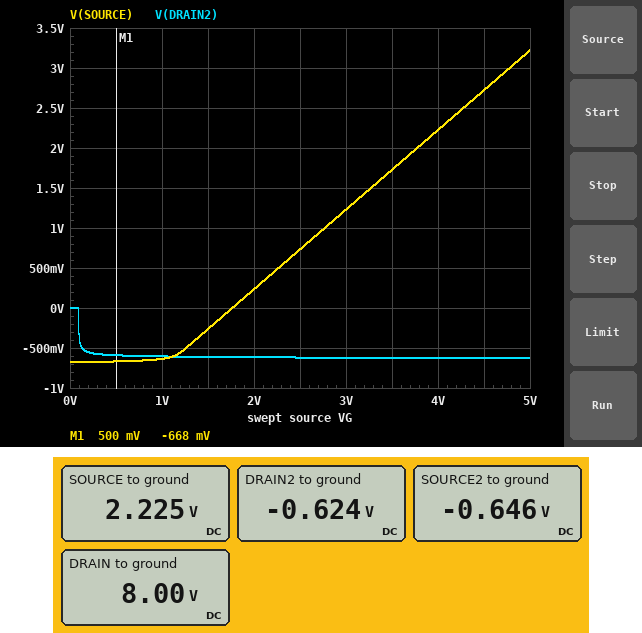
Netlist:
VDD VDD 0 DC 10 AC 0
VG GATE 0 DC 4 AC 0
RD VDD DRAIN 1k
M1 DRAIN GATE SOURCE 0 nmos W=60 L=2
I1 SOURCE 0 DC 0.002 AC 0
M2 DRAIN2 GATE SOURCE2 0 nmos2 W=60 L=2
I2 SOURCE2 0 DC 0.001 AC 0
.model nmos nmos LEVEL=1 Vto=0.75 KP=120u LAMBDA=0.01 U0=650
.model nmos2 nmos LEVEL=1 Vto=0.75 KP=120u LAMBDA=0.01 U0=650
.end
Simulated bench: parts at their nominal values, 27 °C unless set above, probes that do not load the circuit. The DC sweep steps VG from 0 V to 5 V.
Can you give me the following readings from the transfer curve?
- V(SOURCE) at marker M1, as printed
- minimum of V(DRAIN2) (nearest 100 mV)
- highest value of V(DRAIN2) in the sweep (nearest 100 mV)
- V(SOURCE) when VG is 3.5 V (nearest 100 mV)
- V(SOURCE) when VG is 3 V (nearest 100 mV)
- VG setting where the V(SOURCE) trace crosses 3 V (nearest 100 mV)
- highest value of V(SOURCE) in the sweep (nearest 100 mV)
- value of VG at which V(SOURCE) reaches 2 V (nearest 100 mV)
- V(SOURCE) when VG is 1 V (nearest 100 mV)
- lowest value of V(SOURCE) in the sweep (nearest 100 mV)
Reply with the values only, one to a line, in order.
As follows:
-668 mV
-600 mV
0 V
1.7 V
1.2 V
4.8 V
3.2 V
3.8 V
-600 mV
-700 mV
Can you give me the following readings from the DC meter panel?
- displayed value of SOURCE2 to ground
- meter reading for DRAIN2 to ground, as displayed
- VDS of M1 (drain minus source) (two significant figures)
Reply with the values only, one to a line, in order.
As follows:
-0.646 V
-0.624 V
5.8 V
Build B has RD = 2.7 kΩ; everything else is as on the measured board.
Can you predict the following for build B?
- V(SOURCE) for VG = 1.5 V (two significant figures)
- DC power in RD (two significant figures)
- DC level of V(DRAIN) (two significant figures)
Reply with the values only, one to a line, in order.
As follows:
-280 mV
11 mW
4.6 V
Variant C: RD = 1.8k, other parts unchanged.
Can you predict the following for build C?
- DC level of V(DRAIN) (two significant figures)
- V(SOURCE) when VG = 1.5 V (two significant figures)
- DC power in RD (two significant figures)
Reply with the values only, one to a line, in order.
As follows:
6.4 V
-270 mV
7.2 mW
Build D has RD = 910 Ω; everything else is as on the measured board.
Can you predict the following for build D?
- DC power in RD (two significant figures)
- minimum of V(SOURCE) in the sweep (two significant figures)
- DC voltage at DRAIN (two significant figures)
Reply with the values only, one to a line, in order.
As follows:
3.6 mW
-670 mV
8.2 V
